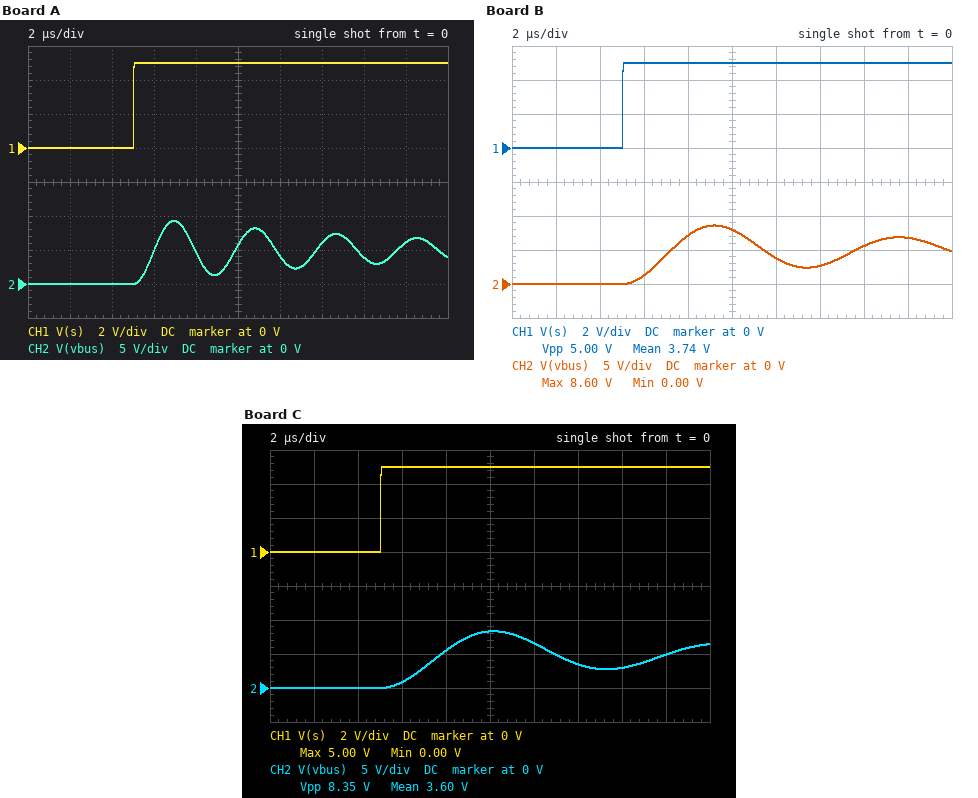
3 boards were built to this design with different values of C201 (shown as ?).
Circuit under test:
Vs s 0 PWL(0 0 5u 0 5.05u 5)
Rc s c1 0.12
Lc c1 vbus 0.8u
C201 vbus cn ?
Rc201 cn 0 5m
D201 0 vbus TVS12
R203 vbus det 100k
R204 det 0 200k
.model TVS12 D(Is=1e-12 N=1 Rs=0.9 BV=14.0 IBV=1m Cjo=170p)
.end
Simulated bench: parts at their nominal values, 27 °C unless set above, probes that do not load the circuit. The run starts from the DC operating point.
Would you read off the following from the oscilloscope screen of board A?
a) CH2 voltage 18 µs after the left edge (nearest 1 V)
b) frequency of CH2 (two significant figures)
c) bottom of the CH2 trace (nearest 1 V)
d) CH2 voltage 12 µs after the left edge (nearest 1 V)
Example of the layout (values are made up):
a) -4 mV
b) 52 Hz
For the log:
a) 6 V
b) 260 kHz
c) 0 V
d) 4 V
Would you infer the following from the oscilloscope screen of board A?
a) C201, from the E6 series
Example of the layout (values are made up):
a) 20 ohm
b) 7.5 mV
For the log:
a) 470 nF
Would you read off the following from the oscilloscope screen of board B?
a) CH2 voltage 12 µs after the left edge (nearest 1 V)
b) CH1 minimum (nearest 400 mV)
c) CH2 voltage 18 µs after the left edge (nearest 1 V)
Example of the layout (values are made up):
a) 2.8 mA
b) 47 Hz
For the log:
a) 4 V
b) 0 V
c) 7 V
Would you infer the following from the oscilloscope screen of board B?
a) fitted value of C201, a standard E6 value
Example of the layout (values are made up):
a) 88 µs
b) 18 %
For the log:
a) 2.2 µF
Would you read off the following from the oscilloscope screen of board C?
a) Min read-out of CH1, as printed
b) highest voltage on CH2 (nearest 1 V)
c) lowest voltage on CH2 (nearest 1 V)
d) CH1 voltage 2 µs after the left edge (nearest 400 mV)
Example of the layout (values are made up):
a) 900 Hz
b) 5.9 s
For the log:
a) 0.00 V
b) 8 V
c) 0 V
d) 0 V
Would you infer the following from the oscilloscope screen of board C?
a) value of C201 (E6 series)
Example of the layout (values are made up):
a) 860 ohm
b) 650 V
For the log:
a) 3.3 µF
